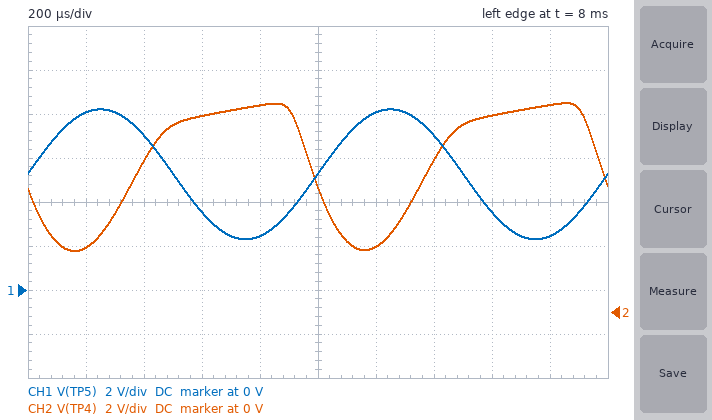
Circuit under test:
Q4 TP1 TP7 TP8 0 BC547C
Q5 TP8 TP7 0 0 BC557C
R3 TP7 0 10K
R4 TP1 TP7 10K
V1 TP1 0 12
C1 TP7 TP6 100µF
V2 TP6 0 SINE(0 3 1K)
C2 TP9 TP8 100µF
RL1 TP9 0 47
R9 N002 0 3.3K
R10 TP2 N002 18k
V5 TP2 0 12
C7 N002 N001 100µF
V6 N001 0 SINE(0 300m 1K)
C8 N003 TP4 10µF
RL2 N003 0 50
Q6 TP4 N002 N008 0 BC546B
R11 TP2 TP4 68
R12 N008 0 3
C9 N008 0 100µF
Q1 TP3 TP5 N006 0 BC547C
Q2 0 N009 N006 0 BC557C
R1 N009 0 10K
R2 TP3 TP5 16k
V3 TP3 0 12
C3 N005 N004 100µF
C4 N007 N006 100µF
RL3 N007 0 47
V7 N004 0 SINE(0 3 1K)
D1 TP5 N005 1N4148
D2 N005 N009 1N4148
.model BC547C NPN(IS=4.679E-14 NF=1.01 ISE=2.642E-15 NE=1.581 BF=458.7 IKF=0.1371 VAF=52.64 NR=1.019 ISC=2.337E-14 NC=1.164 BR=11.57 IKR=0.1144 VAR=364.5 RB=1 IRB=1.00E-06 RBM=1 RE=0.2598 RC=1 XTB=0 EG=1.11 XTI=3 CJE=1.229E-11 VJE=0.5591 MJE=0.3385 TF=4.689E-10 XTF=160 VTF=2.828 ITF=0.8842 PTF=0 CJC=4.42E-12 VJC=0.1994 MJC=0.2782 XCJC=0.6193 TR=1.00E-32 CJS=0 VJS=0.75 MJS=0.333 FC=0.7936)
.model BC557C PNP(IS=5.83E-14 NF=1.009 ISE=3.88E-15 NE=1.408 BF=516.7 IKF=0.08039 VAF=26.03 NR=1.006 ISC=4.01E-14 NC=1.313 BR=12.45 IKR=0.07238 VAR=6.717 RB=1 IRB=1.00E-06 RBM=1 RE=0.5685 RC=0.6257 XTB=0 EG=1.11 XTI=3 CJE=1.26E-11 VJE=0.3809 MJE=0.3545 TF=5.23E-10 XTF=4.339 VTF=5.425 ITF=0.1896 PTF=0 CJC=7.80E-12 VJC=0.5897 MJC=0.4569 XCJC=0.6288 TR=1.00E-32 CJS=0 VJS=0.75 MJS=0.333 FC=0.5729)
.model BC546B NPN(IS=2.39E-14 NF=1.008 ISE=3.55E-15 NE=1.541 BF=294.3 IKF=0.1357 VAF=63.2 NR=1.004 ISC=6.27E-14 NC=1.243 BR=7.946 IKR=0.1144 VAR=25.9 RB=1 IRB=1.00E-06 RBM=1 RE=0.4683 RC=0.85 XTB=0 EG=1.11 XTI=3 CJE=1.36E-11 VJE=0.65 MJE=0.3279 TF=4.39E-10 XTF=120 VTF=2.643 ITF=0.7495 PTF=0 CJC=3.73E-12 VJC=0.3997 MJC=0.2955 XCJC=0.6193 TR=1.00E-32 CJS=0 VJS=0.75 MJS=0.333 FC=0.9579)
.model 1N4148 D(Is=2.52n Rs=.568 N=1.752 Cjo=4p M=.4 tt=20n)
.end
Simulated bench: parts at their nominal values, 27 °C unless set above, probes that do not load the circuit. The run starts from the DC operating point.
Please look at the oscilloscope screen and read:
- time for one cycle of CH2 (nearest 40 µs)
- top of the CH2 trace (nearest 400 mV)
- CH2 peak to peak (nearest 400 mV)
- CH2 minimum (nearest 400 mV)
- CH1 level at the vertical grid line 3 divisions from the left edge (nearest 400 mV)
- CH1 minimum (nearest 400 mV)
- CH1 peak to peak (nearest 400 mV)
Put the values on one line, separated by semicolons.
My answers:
1.00 ms; 9.6 V; 6.8 V; 2.8 V; 3.6 V; 2.4 V; 6.0 V
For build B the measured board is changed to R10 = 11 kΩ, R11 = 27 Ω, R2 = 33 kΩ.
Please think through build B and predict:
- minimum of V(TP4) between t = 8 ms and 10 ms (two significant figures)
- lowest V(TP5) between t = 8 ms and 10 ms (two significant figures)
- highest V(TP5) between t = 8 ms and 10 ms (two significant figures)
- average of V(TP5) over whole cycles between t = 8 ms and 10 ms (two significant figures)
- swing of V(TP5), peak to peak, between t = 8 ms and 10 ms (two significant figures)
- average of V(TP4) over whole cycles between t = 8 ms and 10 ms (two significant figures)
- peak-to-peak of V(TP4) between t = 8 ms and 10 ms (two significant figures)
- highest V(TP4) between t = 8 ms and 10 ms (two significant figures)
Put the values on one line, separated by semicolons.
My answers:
6.2 V; 600 mV; 6.5 V; 3.6 V; 5.9 V; 8.9 V; 4.9 V; 11 V
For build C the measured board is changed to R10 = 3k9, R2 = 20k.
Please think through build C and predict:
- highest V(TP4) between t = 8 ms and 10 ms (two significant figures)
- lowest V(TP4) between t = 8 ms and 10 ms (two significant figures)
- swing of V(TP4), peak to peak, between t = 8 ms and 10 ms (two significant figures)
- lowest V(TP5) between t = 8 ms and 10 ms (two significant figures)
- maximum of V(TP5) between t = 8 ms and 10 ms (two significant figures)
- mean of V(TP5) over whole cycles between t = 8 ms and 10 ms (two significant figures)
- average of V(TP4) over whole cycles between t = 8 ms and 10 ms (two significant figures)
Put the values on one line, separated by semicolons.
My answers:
8.1 V; 780 mV; 7.3 V; 1.7 V; 7.6 V; 4.7 V; 4.6 V
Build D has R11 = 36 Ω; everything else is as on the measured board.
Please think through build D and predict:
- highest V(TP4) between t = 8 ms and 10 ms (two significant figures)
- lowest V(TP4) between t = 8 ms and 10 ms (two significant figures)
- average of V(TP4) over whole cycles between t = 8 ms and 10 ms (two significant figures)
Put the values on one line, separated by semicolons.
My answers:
11 V; 6.2 V; 9.2 V
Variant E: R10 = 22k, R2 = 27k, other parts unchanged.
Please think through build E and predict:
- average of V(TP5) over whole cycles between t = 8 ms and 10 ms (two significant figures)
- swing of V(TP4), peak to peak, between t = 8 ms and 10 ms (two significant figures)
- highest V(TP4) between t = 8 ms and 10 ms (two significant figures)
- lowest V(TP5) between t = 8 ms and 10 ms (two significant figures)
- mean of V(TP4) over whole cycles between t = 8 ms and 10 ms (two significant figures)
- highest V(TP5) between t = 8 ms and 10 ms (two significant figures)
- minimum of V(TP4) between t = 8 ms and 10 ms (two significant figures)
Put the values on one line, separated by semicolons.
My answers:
4.0 V; 6.2 V; 9.9 V; 1.0 V; 7.6 V; 6.9 V; 3.7 V
